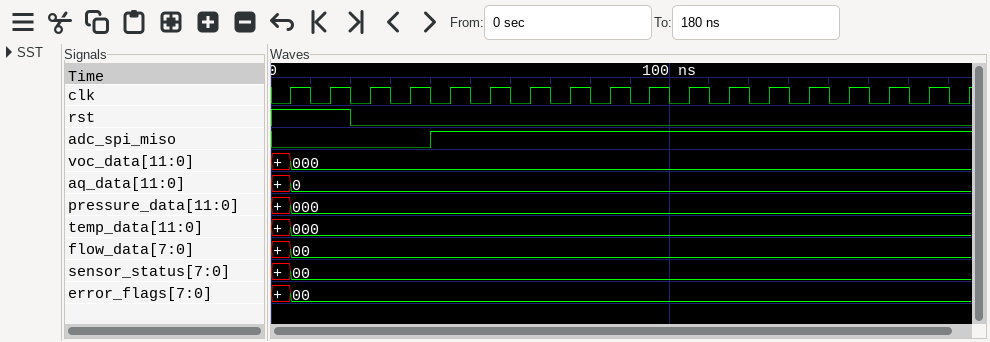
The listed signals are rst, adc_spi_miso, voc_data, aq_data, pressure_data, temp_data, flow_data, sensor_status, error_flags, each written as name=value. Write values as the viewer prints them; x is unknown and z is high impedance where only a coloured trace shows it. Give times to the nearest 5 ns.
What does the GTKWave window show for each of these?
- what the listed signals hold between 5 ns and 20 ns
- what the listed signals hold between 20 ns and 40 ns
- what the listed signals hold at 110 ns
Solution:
rst=1, adc_spi_miso=0, voc_data=000, aq_data=0, pressure_data=000, temp_data=000, flow_data=00, sensor_status=00, error_flags=00
rst=0, adc_spi_miso=0, voc_data=000, aq_data=0, pressure_data=000, temp_data=000, flow_data=00, sensor_status=00, error_flags=00
rst=0, adc_spi_miso=1, voc_data=000, aq_data=0, pressure_data=000, temp_data=000, flow_data=00, sensor_status=00, error_flags=00
